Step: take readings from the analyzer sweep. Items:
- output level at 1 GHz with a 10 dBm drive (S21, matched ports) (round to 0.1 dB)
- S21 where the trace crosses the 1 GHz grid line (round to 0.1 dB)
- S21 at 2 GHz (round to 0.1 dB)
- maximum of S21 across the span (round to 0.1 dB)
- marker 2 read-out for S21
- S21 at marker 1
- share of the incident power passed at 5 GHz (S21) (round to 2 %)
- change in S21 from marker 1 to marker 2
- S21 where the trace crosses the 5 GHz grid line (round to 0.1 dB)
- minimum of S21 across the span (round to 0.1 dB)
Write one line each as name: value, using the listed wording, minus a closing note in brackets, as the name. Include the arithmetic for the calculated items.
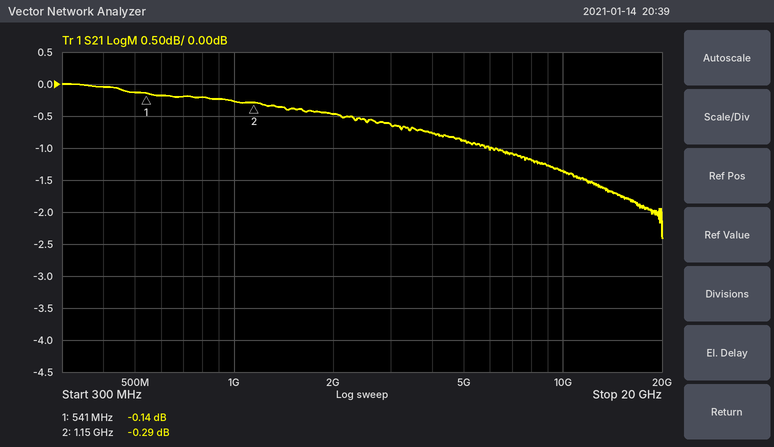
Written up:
output level at 1 GHz with a 10 dBm drive (S21, matched ports): 10 dBm + (-0.3 dB) = 9.7 dBm
S21 where the trace crosses the 1 GHz grid line: -0.3 dB
S21 at 2 GHz: -0.5 dB
maximum of S21 across the span: 0.0 dB
marker 2 read-out for S21: -0.29 dB
S21 at marker 1: -0.14 dB
share of the incident power passed at 5 GHz (S21): 10^(-0.9/10) ≈ 81.3 %, so 82 % to the nearest 2 %
change in S21 from marker 1 to marker 2: -0.29 − (-0.14) = -0.15 dB
S21 where the trace crosses the 5 GHz grid line: -0.9 dB
minimum of S21 across the span: -2.4 dB
